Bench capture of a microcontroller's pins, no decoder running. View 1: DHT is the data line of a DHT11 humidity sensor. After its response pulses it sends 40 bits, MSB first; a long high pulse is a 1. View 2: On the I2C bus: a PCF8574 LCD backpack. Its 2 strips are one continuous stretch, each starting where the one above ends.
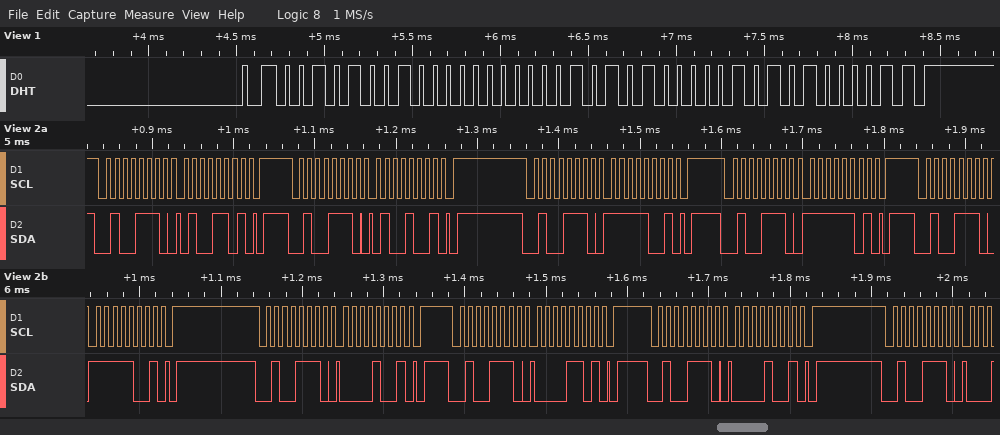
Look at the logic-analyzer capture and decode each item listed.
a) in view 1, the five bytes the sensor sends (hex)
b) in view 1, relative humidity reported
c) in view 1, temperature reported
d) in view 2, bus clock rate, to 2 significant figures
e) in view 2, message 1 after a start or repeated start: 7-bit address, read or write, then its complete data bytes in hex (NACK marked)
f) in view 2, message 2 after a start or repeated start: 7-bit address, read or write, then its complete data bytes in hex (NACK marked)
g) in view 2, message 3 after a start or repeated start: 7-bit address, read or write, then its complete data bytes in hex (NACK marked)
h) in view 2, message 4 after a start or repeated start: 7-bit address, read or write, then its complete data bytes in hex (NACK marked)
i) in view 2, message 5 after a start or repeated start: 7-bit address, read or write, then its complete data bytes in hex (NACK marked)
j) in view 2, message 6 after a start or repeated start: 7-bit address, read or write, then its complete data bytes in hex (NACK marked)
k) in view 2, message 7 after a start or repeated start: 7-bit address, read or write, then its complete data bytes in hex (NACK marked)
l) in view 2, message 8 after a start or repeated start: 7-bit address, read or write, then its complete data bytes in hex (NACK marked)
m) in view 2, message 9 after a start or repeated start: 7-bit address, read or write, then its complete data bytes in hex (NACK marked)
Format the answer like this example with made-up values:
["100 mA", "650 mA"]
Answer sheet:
["29 00 15 05 43", "41 %", "21.5 °C", "100 kHz", "0x27 write: 4D", "0x27 write: 49", "0x27 write: F9", "0x27 write: FD", "0x27 write: F9", "0x27 write: 09", "0x27 write: 0D", "0x27 write: 09", "0x27 write"]
